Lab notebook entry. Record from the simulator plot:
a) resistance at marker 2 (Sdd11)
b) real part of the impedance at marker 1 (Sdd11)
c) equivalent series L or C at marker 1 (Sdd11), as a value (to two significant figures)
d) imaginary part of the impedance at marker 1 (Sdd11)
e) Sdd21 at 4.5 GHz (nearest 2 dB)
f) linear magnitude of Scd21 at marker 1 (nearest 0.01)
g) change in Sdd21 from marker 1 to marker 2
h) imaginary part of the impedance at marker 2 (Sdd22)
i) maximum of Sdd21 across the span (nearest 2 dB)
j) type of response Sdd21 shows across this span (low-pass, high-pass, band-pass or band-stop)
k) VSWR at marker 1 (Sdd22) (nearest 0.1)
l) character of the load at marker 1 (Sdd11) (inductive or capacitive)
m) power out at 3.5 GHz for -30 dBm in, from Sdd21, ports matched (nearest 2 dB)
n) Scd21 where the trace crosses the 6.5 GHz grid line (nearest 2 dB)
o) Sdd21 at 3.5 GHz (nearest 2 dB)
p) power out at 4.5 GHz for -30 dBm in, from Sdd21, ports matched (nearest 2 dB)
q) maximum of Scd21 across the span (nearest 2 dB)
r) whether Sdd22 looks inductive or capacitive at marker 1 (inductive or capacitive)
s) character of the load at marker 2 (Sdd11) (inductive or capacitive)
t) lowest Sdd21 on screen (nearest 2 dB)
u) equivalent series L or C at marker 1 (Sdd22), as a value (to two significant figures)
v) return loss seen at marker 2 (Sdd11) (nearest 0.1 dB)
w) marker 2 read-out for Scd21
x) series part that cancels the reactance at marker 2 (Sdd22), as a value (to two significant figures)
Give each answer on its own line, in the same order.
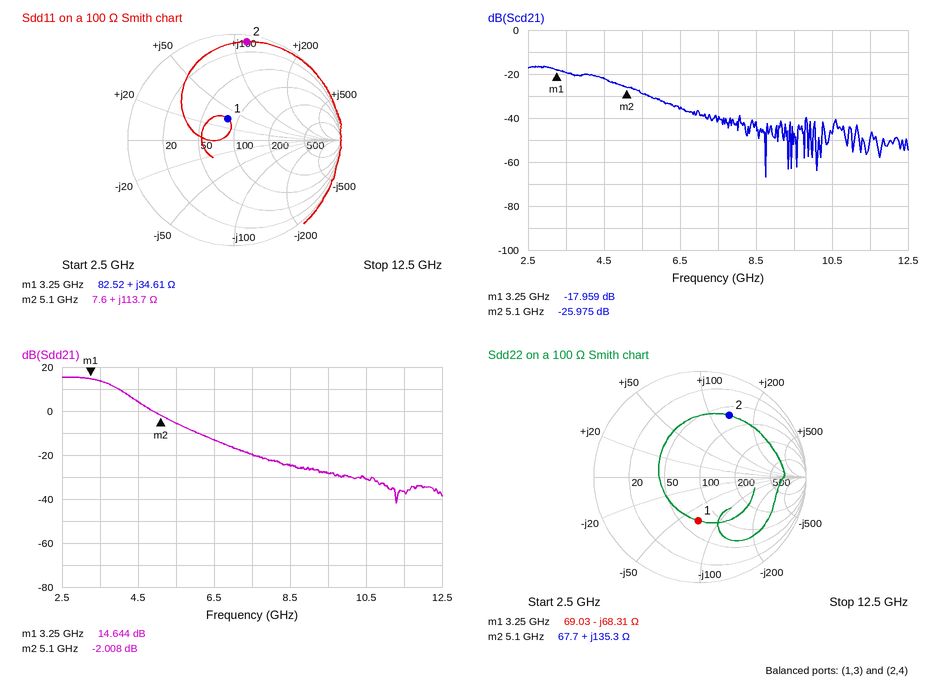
7.6 Ω
82.52 Ω
1.7 nH
+34.61 Ω
4 dB
0.13
-16.652 dB
+135.3 Ω
16 dB
low-pass
2.4
inductive
-16 dBm
-36 dB
14 dB
-26 dBm
-16 dB
capacitive
inductive
-42 dB
720 fF
0.6 dB
-25.975 dB
230 fF
